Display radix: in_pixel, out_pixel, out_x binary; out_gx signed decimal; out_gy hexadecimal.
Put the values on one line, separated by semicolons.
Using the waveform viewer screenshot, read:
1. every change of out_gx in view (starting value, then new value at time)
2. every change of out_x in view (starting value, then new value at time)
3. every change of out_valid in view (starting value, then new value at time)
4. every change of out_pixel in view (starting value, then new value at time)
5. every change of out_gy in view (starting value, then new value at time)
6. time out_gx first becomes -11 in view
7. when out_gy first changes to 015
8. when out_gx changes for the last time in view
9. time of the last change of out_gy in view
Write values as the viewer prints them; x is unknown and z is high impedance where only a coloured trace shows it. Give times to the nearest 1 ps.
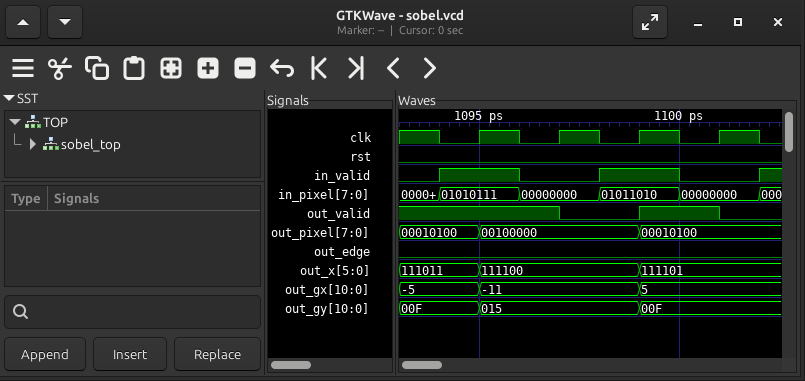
-5, -11 at 1095 ps, 5 at 1099 ps; 111011, 111100 at 1095 ps, 111101 at 1099 ps; 1, 0 at 1097 ps, 1 at 1099 ps, 0 at 1101 ps; 00010100, 00100000 at 1095 ps, 00010100 at 1099 ps; 00F, 015 at 1095 ps, 00F at 1099 ps; 1095 ps; 1095 ps; 1099 ps; 1099 ps
